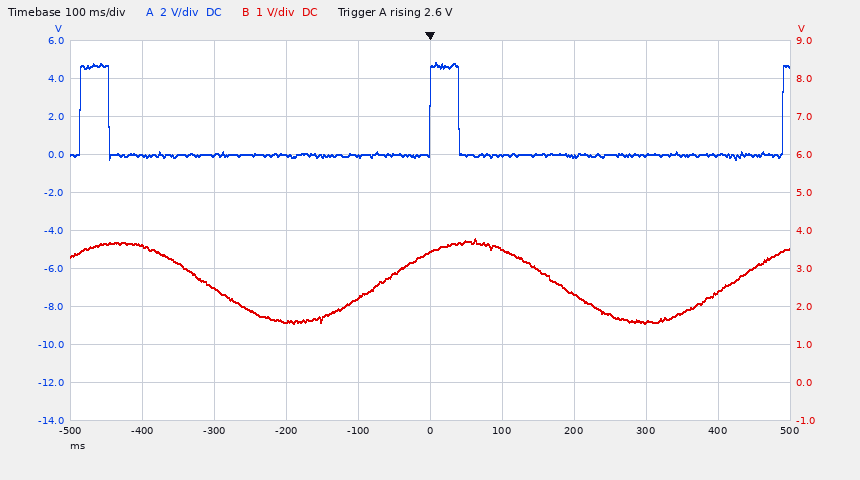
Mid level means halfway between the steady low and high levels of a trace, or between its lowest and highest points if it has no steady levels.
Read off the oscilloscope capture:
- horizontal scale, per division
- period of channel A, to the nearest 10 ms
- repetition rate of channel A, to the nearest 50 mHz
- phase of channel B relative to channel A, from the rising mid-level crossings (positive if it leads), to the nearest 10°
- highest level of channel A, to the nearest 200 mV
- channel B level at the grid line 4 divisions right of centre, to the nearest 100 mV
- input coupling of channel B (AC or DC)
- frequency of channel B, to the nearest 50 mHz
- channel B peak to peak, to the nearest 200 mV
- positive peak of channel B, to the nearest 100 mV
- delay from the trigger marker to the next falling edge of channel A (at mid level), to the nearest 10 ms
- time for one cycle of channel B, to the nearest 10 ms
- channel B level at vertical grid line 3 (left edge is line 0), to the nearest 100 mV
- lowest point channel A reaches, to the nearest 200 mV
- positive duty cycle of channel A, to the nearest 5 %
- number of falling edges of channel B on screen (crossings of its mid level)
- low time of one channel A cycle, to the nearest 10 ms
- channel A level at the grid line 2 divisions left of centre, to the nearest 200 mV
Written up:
100 ms
490 ms
2.05 Hz
+50°
4.8 V
2.4 V
DC
2.05 Hz
2.2 V
3.8 V
40 ms
490 ms
1.6 V
-200 mV
10 %
2
450 ms
0.0 V
